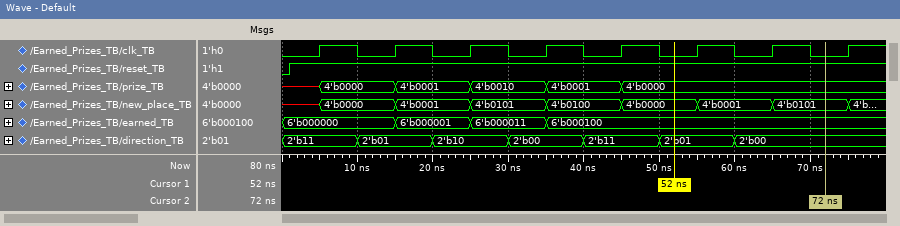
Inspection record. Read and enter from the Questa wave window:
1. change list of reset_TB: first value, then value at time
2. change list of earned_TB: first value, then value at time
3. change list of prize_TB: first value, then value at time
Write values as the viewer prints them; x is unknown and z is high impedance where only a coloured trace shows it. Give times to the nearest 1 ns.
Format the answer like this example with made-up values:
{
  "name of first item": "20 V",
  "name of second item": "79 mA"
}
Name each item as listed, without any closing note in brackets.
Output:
{
  "change list of reset_TB: first value, then value at time": "0, 1 at 1 ns",
  "change list of earned_TB: first value, then value at time": "6'b000000, 6'b000001 at 15 ns, 6'b000011 at 25 ns, 6'b000100 at 35 ns",
  "change list of prize_TB: first value, then value at time": "x, 4'b0000 at 5 ns, 4'b0001 at 15 ns, 4'b0010 at 25 ns, 4'b0001 at 35 ns, 4'b0000 at 45 ns"
}
